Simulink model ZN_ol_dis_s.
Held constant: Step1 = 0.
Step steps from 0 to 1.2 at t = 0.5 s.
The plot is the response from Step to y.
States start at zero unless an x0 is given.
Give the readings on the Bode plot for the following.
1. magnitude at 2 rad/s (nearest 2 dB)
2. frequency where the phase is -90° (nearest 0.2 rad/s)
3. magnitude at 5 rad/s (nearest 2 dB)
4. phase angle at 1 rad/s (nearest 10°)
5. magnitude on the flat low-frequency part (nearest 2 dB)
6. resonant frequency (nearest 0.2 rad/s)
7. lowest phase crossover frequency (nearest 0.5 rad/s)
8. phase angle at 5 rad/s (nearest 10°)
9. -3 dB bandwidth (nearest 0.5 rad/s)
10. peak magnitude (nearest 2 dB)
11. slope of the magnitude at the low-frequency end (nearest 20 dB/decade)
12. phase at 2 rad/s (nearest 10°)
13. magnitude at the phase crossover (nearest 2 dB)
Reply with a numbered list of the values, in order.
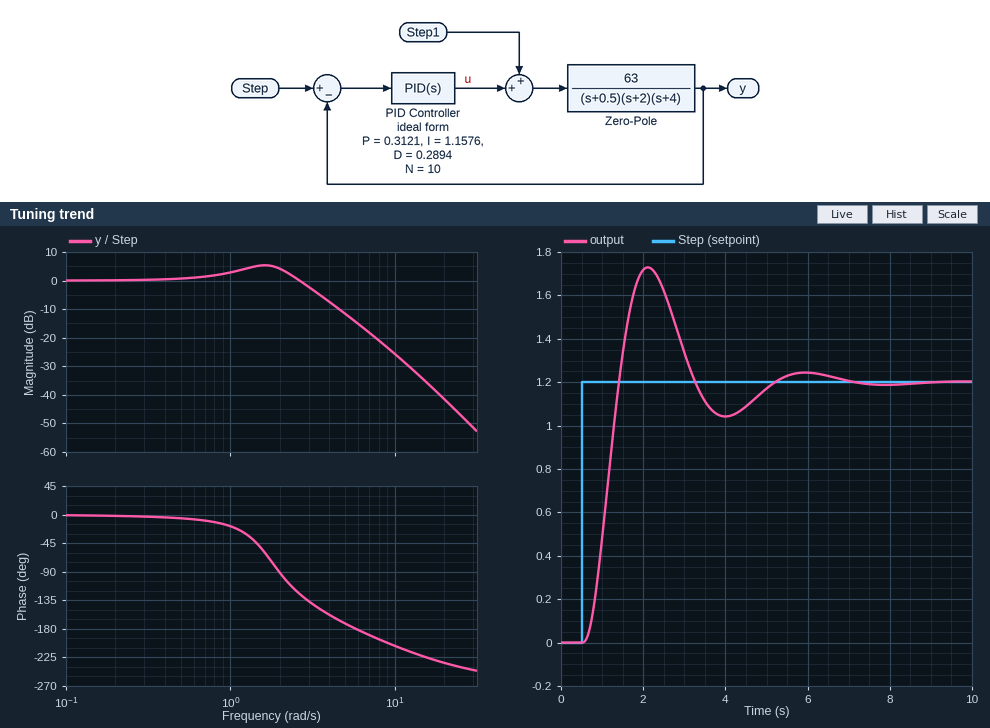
1. 4 dB
2. 2.0 rad/s
3. -12 dB
4. -20°
5. 0 dB
6. 1.6 rad/s
7. 6.0 rad/s
8. -170°
9. 3.0 rad/s
10. 6 dB
11. 0 dB/decade
12. -90°
13. -14 dB
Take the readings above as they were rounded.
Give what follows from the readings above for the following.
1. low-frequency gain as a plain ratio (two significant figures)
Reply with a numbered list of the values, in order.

1. 1.0
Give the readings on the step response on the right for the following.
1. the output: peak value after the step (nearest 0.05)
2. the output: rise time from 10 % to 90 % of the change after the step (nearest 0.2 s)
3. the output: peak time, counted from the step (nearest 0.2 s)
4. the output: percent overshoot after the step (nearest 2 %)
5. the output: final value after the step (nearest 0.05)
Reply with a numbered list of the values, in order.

1. 1.75
2. 0.6 s
3. 1.6 s
4. 44 %
5. 1.20
